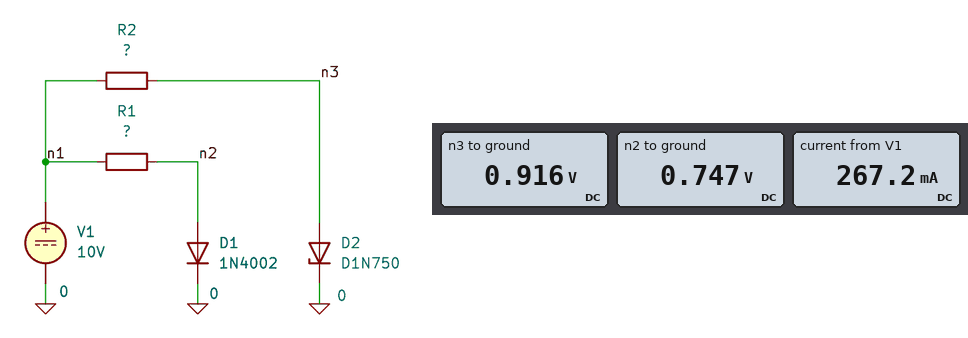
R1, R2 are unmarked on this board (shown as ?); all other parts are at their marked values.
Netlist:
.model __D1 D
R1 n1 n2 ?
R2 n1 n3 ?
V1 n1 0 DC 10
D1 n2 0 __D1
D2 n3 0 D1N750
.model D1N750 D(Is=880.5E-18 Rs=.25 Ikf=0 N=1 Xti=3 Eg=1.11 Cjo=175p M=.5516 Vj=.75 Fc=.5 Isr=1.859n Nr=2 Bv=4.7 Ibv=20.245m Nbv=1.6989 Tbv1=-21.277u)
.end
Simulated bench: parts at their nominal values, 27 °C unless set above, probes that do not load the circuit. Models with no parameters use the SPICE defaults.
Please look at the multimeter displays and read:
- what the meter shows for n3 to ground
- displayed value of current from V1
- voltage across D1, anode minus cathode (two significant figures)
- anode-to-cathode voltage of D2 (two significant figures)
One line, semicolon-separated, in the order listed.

0.916 V; 267.2 mA; 750 mV; 920 mV
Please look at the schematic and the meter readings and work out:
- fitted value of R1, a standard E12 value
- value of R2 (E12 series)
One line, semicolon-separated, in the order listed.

270 Ω; 39 Ω
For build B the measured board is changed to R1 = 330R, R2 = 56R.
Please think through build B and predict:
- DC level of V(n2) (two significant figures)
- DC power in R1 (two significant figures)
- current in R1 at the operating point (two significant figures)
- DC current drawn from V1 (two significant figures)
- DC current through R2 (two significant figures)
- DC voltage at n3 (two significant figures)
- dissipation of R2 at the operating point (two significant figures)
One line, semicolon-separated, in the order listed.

740 mV; 260 mW; 28 mA; 190 mA; 160 mA; 890 mV; 1.5 W
